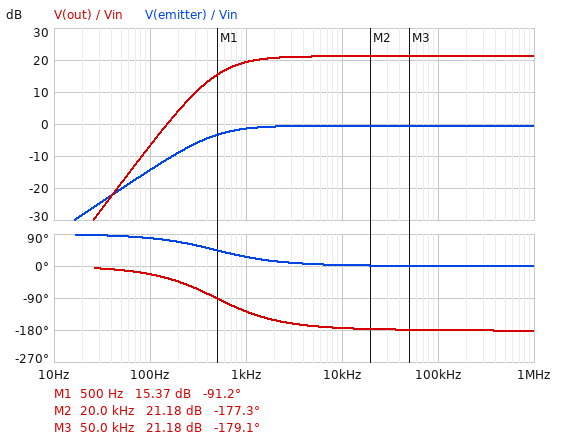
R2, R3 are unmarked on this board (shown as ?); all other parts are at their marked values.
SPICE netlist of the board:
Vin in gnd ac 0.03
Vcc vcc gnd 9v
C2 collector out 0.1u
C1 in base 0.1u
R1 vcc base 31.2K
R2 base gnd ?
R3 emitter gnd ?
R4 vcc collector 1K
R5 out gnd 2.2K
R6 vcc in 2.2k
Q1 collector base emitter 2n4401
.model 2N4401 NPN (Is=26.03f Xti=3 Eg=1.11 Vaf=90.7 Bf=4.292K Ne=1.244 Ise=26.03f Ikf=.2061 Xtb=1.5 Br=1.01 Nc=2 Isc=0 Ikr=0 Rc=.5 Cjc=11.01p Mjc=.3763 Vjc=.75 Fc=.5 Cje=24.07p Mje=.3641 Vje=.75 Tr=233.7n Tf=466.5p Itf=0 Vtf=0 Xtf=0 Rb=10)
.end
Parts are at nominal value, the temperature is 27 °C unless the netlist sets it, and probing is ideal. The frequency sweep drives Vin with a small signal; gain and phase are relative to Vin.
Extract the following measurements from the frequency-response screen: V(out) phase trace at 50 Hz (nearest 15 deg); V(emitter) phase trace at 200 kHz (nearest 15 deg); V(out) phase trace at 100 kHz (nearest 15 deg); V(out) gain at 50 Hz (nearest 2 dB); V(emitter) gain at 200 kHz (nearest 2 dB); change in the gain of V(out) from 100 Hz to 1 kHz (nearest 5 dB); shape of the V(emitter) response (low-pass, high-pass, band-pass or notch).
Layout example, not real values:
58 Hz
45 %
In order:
-15 deg
0 deg
-180 deg
-18 dB
0 dB
25 dB
high-pass
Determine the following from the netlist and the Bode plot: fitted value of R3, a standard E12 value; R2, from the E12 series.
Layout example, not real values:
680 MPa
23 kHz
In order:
56 Ω
5.6 kΩ
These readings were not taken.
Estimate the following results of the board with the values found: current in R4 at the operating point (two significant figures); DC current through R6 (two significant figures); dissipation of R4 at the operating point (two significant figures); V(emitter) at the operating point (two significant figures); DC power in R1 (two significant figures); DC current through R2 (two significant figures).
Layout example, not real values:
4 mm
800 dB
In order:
8.1 mA
4.1 mA
65 mW
450 mV
2.0 mW
200 µA
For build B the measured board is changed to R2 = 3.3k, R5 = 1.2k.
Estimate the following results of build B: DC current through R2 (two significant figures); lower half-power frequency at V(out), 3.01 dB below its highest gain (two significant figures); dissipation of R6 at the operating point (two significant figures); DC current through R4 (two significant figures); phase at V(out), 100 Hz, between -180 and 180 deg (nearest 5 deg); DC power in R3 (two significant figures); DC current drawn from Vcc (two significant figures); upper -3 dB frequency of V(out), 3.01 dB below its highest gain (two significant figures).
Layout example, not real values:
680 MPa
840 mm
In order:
240 µA
1.1 kHz
37 mW
2.7 mA
-15 deg
410 µW
7.0 mA
49 MHz
